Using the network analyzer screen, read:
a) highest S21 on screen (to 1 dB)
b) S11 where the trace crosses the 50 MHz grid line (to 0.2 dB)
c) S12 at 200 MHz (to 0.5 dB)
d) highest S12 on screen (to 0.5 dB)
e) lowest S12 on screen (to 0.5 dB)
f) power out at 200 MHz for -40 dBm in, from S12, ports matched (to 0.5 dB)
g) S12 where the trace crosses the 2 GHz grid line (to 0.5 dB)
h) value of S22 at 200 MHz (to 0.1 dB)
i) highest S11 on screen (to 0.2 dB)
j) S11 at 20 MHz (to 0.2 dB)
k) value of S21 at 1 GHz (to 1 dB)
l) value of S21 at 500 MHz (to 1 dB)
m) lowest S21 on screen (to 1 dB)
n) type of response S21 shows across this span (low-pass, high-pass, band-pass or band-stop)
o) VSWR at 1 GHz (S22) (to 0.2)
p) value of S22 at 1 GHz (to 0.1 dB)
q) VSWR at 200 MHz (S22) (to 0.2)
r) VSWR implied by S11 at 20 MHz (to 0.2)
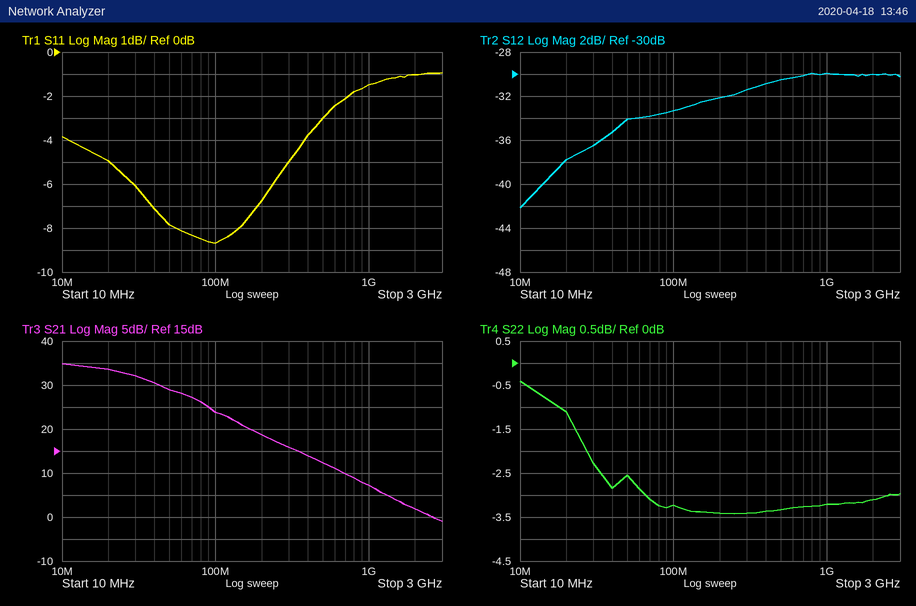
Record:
35 dB
-7.8 dB
-32.0 dB
-30.0 dB
-42.0 dB
-72.0 dBm
-30.0 dB
-3.4 dB
-1.0 dB
-5.0 dB
7 dB
12 dB
-1 dB
low-pass
5.4
-3.2 dB
5.2
3.6
